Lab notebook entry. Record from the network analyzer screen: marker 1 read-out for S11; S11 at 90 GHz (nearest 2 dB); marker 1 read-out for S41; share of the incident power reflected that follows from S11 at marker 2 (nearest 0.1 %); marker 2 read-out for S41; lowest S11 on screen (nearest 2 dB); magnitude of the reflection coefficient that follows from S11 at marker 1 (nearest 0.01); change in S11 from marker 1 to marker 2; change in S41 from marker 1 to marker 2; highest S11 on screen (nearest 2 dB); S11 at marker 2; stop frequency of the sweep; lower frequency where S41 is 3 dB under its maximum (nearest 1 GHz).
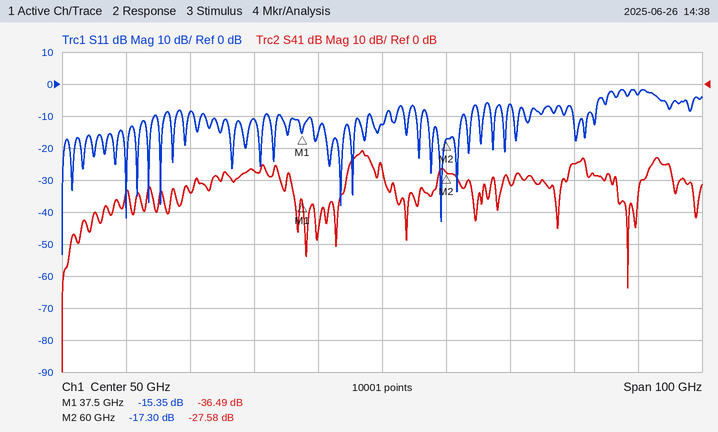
-15.35 dB
-4 dB
-36.49 dB
1.9 %
-27.58 dB
-54 dB
0.17
-1.95 dB
8.91 dB
-2 dB
-17.30 dB
100 GHz
45 GHz
